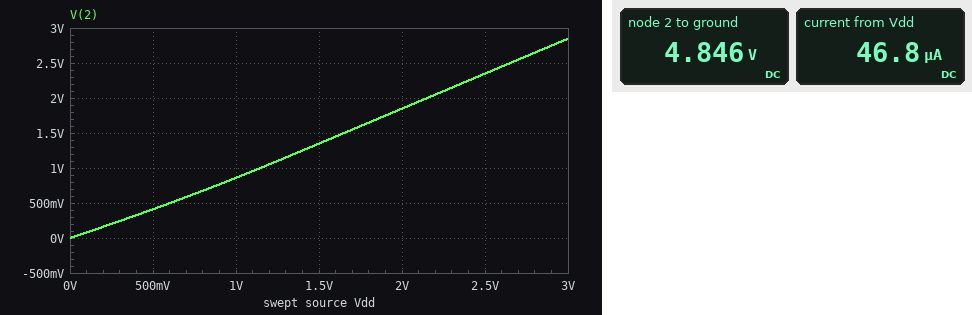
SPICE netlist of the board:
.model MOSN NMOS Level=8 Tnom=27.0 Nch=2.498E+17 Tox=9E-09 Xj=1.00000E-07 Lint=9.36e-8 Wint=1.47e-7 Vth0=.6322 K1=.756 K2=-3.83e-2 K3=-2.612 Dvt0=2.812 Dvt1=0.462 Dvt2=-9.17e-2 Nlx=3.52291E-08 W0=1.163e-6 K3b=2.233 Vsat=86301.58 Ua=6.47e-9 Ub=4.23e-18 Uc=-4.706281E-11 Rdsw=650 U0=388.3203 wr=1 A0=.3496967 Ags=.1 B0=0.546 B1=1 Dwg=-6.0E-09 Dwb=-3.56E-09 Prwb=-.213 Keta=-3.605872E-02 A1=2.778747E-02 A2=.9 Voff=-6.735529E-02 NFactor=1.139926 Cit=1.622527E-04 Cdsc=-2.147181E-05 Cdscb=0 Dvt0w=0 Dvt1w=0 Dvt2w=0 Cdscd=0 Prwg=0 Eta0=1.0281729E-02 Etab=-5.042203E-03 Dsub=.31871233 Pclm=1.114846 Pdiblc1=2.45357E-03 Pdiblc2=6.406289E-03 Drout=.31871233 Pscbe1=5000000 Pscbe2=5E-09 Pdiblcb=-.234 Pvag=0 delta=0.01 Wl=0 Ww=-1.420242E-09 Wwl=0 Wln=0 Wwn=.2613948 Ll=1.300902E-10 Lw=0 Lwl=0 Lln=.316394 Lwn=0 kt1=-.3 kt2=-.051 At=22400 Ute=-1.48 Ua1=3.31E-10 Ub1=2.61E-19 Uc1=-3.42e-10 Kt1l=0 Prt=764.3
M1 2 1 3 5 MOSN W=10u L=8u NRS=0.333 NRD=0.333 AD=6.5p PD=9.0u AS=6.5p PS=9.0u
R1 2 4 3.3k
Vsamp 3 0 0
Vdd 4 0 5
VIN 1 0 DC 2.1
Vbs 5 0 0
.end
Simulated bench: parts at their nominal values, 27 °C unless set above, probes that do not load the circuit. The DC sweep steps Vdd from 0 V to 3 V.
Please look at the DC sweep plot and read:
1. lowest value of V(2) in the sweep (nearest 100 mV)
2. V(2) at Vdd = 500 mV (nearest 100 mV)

0 V
400 mV
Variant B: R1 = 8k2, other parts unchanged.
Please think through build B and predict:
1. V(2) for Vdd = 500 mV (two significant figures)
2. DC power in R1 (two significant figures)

320 mV
18 µW
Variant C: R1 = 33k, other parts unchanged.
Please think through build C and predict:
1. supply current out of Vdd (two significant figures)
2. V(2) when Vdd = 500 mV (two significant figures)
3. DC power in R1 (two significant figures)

46 µA
140 mV
71 µW
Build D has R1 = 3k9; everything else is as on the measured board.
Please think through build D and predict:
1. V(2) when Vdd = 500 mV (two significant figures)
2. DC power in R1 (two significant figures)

400 mV
8.5 µW
